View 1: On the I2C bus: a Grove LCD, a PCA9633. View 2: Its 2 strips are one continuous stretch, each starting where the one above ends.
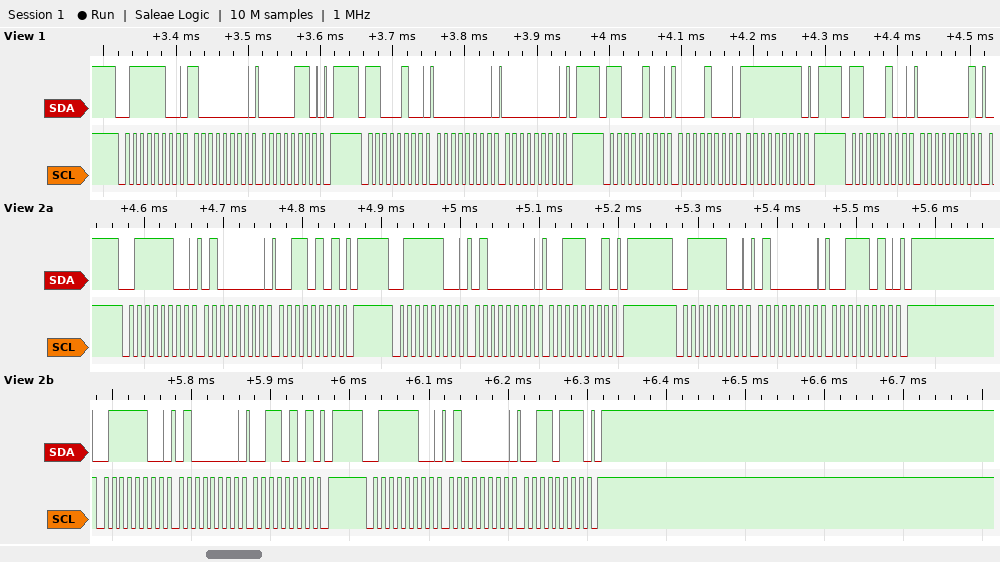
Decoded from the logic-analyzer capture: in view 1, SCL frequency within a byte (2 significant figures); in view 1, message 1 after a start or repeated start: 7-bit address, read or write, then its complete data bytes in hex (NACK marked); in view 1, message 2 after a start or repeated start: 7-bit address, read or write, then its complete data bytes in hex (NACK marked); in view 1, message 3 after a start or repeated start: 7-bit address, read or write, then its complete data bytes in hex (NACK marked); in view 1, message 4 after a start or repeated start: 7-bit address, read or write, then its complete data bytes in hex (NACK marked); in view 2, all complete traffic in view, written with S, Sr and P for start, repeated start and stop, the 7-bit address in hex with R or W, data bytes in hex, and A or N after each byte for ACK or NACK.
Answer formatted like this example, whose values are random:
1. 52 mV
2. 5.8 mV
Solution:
1. 100 kHz
2. 0x3E write: 80 06
3. 0x62 write: 00 00
4. 0x62 write: 08 FF
5. 0x62 write: 01
6. S 3EW A 40 A 35 A P S 3EW A 40 A 39 A P S 3EW A 40 A 3A A P S 3EW A 40 A 35 A P S 3EW A 40 A 37 A P
